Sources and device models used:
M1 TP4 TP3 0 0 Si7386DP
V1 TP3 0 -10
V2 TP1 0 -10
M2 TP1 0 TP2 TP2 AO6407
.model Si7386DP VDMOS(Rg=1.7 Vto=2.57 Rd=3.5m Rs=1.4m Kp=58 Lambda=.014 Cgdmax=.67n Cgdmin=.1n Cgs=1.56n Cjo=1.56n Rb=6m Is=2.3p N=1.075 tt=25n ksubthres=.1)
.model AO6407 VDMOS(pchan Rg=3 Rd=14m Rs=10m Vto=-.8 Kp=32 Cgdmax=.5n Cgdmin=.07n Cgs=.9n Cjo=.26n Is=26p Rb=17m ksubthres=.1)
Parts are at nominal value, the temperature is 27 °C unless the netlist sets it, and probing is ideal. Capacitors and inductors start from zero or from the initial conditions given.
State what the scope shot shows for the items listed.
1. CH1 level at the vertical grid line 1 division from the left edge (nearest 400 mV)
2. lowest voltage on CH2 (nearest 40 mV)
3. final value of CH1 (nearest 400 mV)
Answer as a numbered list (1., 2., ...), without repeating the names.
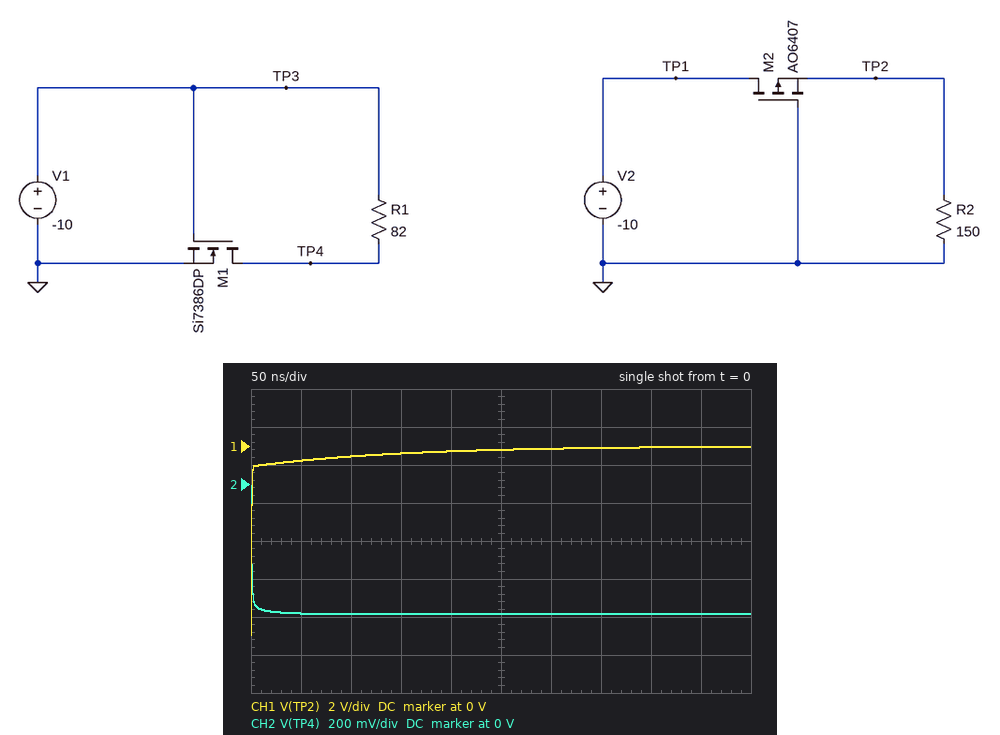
1. -800 mV
2. -680 mV
3. 0 V
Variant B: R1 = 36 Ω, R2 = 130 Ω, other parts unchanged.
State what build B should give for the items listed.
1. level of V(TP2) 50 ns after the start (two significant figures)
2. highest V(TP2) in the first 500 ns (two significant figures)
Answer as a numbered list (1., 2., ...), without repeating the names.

1. -730 mV
2. -22 mV
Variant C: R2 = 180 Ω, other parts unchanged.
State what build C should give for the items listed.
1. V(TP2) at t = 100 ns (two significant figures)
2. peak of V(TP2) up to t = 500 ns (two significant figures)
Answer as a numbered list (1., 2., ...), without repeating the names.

1. -620 mV
2. -65 mV
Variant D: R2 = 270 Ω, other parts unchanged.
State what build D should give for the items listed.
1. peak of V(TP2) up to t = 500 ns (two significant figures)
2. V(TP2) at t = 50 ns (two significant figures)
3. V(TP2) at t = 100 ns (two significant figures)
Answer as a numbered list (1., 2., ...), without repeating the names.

1. -170 mV
2. -920 mV
3. -760 mV
